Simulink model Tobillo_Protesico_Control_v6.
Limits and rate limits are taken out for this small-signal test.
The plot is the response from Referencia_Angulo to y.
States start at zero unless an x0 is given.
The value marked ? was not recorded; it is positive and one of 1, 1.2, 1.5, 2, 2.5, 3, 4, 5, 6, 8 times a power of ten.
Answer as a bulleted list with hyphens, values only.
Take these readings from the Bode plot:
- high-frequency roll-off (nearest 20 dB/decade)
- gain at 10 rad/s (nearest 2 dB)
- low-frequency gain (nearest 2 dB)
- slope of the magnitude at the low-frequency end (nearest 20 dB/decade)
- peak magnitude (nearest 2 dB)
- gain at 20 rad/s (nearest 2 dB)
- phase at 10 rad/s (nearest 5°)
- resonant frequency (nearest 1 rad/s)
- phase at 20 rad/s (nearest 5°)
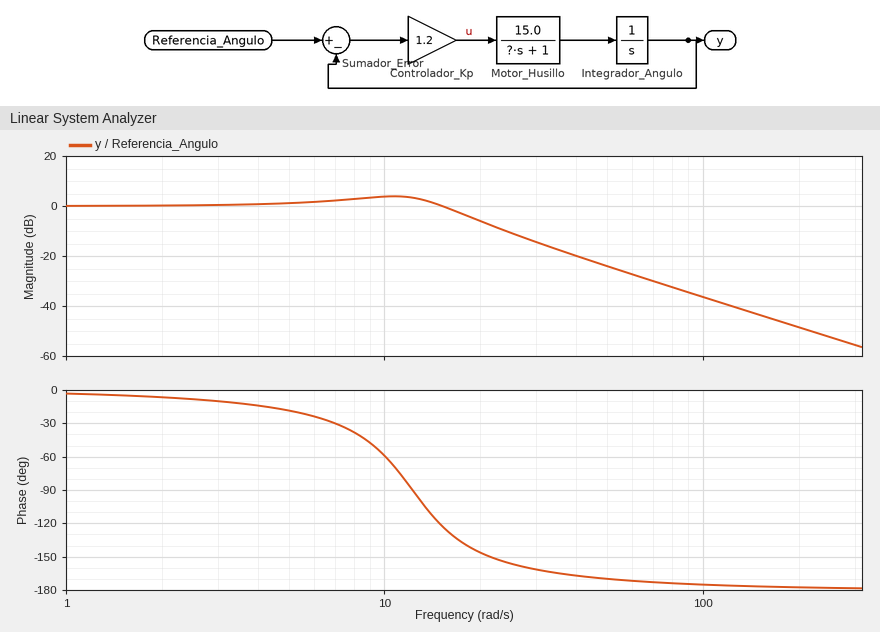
- -40 dB/decade
- 4 dB
- 0 dB
- 0 dB/decade
- 4 dB
- -6 dB
- -60°
- 11 rad/s
- -145°
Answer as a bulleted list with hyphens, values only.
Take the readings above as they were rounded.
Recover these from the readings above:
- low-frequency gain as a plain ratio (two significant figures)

- 1.0
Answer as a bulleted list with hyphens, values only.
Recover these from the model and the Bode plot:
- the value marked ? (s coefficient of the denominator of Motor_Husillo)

- 0.12
